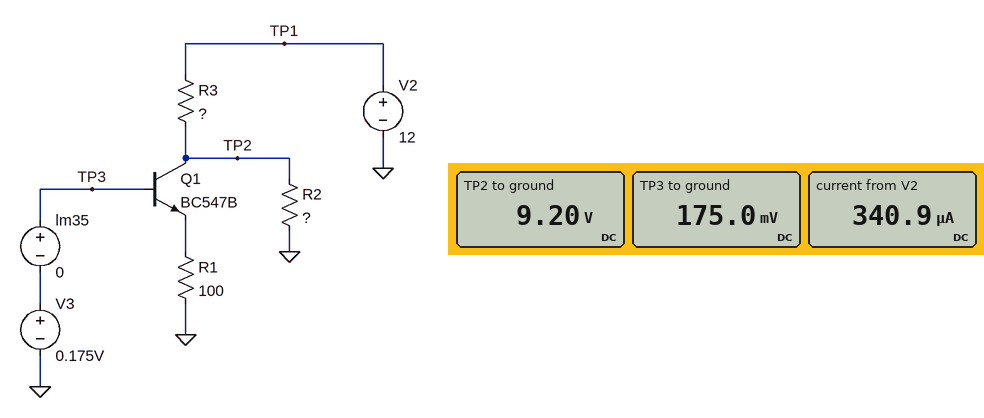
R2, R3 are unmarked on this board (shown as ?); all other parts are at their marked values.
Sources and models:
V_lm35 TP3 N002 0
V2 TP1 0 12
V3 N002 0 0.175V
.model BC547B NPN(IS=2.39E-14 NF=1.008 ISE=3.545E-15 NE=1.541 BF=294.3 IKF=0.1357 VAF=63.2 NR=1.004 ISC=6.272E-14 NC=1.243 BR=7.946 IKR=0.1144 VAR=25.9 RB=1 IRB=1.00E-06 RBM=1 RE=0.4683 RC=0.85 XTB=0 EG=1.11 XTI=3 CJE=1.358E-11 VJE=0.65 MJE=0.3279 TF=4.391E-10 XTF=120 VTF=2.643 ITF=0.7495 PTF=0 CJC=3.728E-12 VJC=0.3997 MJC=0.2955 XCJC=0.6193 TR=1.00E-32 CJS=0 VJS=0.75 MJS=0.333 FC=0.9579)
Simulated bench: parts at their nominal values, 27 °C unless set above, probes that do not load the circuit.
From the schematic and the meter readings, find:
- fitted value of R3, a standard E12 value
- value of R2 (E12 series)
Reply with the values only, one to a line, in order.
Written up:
8.2 kΩ
27 kΩ
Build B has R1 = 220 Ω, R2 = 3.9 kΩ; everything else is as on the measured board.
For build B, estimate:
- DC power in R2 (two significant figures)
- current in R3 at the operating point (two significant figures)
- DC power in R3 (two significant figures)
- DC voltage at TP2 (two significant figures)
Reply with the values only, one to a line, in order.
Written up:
3.8 mW
990 µA
8.1 mW
3.9 V
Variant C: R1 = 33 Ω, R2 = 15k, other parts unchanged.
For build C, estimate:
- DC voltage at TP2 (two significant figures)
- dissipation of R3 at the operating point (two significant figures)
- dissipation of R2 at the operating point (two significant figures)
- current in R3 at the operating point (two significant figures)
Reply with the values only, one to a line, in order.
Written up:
7.8 V
2.2 mW
4.0 mW
520 µA
